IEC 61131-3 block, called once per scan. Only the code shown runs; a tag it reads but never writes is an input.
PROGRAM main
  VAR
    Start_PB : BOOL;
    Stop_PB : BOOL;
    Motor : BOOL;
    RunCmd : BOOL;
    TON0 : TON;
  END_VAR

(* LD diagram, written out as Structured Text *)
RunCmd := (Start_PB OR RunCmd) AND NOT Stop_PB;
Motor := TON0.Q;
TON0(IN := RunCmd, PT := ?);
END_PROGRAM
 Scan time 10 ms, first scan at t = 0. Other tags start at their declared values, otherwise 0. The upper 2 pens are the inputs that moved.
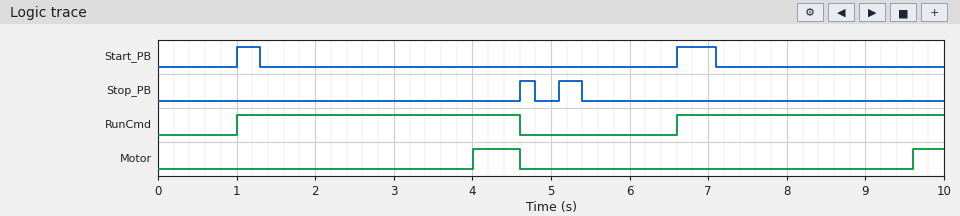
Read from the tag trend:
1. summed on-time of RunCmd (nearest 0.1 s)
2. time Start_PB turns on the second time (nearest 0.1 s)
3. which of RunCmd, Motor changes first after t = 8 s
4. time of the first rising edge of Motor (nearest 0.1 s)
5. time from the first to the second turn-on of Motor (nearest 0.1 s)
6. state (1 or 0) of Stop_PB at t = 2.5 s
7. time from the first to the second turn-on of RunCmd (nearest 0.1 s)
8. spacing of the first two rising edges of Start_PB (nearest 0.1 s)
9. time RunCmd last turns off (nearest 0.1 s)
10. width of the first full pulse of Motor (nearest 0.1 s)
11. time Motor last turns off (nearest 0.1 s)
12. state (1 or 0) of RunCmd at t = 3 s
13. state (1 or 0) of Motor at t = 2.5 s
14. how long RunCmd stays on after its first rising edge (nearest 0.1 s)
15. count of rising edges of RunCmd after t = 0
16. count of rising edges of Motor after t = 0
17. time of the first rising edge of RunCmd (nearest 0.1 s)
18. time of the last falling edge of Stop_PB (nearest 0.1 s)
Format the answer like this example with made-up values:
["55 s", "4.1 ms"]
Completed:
["7.0 s", "6.6 s", "Motor", "4.0 s", "5.6 s", "0", "5.6 s", "5.6 s", "4.6 s", "0.6 s", "4.6 s", "1", "0", "3.6 s", "2", "2", "1.0 s", "5.4 s"]
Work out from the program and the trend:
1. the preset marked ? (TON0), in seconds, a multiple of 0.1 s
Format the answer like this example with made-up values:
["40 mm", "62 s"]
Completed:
["3.0 s"]
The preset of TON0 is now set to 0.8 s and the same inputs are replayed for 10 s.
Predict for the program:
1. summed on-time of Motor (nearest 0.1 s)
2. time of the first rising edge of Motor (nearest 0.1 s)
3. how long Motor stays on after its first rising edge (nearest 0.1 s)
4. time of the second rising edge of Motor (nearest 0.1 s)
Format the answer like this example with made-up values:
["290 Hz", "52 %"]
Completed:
["5.4 s", "1.8 s", "2.8 s", "7.4 s"]
